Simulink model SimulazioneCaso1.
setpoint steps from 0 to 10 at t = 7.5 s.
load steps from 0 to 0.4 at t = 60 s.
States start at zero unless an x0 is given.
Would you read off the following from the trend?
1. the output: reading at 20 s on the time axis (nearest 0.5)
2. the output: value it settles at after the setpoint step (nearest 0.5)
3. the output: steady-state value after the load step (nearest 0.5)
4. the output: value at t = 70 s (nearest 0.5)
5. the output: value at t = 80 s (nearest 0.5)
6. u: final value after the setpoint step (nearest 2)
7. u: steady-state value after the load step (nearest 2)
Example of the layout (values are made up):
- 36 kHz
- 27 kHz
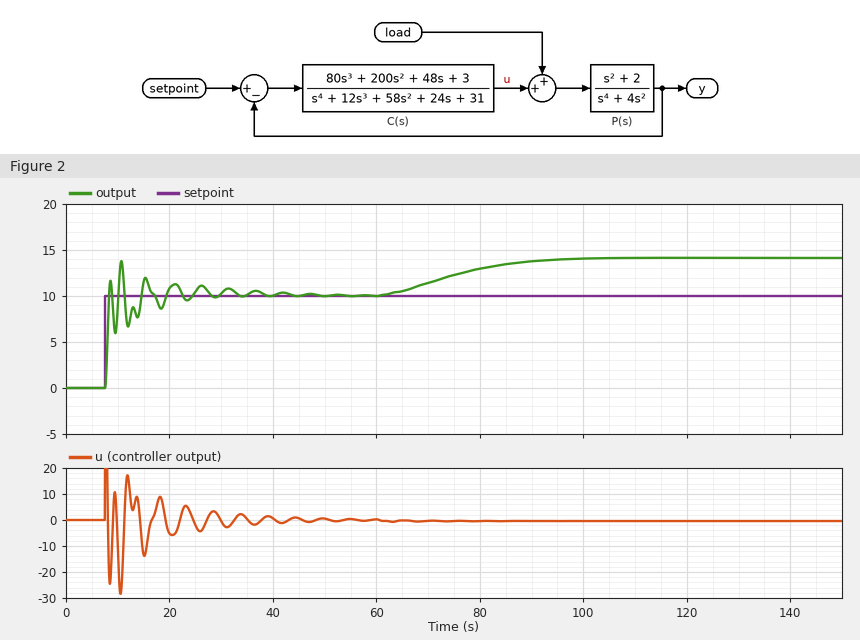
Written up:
- 11.0
- 10.0
- 14.0
- 11.5
- 13.0
- 0
- 0
